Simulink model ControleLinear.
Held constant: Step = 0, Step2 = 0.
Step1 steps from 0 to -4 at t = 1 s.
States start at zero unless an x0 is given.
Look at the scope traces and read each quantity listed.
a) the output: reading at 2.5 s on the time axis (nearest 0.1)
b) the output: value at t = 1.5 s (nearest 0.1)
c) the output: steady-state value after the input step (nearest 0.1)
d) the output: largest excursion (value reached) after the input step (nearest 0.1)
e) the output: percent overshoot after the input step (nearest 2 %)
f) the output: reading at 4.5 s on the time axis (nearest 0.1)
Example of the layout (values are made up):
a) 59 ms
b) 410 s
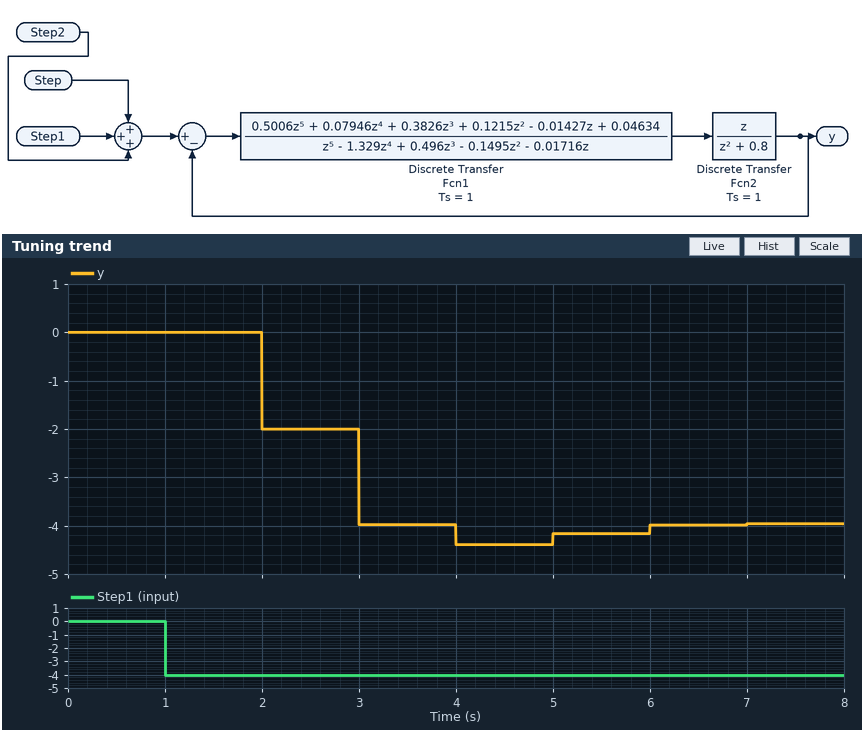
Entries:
a) -2.0
b) 0.0
c) -4.0
d) -4.4
e) 10 %
f) -4.4
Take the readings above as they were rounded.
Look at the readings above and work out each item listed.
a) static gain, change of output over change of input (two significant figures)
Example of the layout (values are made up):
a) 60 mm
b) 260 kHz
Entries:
a) 1.0
